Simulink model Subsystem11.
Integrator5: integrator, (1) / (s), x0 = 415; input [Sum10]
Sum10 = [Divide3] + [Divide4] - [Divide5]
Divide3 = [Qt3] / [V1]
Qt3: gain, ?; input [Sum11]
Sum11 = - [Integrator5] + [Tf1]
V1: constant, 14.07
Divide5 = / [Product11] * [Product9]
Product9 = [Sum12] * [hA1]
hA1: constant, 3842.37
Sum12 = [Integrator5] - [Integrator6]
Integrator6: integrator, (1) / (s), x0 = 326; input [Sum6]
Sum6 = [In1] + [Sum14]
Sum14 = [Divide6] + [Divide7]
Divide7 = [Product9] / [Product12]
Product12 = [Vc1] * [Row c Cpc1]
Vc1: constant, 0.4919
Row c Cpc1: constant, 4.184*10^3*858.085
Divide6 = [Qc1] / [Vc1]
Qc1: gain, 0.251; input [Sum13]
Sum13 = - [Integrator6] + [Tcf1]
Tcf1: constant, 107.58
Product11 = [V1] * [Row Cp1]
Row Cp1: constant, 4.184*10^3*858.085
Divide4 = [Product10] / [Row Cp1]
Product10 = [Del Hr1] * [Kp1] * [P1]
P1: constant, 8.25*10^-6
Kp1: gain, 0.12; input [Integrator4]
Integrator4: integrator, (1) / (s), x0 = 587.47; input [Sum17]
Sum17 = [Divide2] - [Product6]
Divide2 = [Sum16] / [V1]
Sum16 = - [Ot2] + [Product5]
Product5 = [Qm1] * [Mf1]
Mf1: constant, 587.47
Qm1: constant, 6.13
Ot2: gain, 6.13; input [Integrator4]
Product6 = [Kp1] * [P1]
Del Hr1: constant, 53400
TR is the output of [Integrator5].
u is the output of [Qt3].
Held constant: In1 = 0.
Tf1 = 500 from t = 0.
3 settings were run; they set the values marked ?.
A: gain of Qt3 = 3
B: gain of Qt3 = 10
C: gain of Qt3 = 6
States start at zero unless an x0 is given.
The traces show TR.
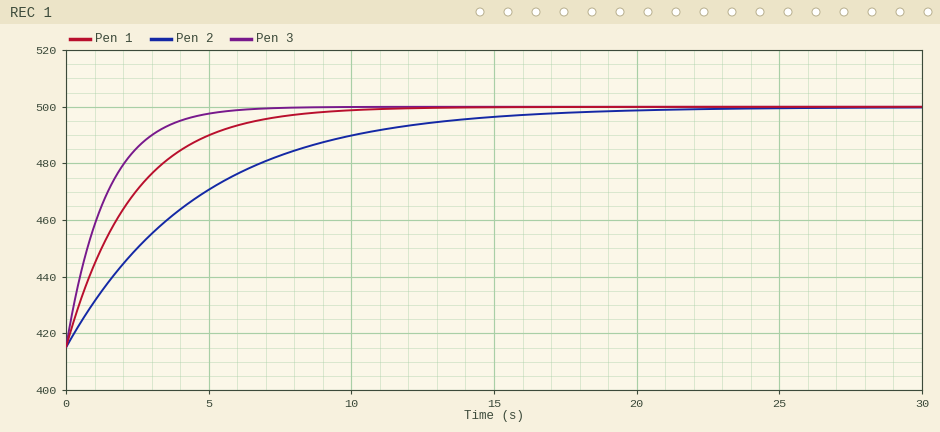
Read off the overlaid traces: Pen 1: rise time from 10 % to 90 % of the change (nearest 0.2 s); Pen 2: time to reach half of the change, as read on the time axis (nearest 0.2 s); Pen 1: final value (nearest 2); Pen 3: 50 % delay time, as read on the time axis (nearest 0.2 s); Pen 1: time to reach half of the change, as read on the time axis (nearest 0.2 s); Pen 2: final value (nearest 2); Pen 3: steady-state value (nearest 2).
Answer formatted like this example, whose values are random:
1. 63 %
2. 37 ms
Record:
1. 5.2 s
2. 3.2 s
3. 500
4. 1.0 s
5. 1.6 s
6. 500
7. 500
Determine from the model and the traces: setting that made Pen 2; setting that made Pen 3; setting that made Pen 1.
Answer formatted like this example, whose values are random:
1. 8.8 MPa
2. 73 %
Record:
1. A
2. B
3. C
